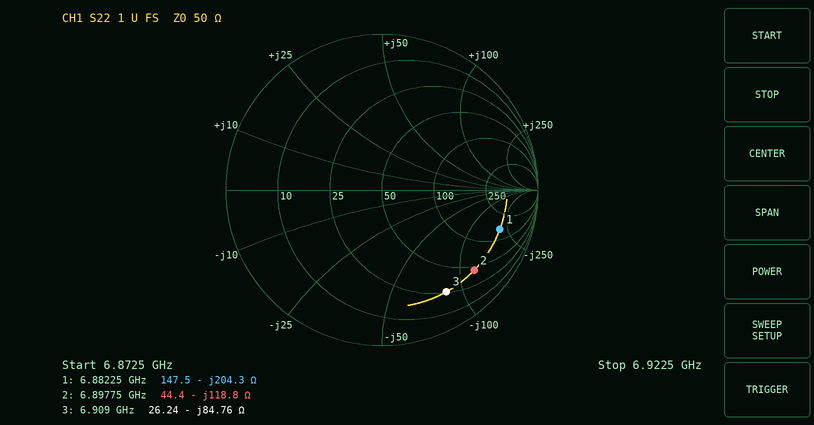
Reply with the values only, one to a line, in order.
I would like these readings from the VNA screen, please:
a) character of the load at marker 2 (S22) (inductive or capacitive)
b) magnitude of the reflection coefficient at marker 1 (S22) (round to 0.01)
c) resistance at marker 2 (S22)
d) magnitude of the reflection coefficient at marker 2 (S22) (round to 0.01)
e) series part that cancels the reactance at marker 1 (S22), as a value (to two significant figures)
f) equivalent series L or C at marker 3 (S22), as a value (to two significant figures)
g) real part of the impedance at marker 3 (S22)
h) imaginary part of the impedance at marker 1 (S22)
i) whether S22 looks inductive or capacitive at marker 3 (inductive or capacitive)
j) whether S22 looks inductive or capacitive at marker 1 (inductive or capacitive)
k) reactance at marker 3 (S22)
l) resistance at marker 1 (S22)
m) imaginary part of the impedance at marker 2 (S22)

capacitive
0.80
44.4 Ω
0.78
4.7 nH
270 fF
26.24 Ω
-204.3 Ω
capacitive
capacitive
-84.76 Ω
147.5 Ω
-118.8 Ω
